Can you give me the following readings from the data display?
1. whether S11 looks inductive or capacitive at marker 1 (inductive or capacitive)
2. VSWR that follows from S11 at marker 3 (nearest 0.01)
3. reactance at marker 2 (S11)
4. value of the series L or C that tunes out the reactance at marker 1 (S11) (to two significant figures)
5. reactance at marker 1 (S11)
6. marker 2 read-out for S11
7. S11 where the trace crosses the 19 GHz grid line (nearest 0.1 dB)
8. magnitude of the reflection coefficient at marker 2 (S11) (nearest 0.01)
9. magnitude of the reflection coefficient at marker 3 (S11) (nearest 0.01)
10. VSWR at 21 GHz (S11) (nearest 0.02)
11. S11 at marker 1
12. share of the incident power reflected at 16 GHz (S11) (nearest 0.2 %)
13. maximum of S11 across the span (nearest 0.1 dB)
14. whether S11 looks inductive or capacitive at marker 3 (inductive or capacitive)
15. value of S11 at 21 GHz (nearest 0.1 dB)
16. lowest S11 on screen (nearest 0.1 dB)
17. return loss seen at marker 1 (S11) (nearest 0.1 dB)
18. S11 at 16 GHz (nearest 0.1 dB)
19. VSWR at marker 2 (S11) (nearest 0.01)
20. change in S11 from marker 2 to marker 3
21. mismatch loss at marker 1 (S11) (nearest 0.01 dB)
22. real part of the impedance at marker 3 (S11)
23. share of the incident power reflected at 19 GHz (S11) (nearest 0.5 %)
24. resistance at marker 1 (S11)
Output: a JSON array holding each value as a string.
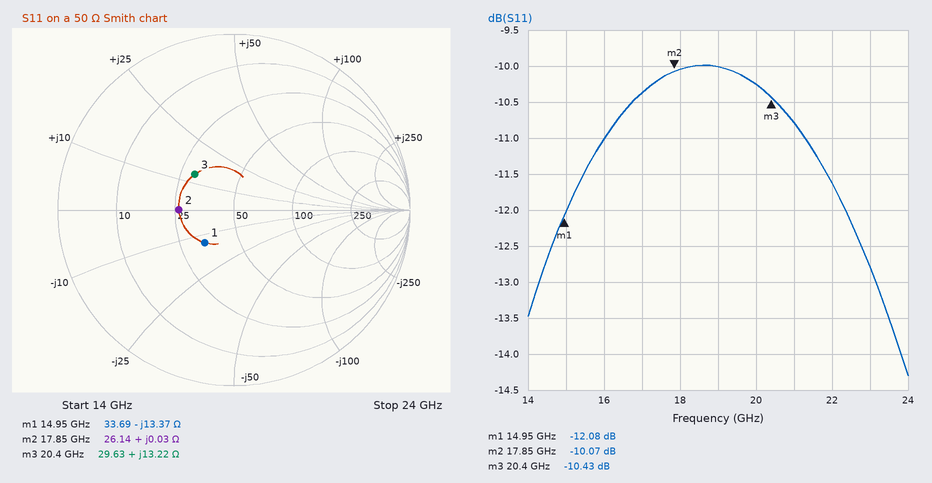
["capacitive", "1.86", "+0.03 Ω", "140 pH", "-13.37 Ω", "-10.07 dB", "-10.0 dB", "0.31", "0.30", "1.82", "-12.08 dB", "8.0 %", "-10.0 dB", "inductive", "-10.8 dB", "-14.3 dB", "12.1 dB", "-11.0 dB", "1.91", "-0.36 dB", "0.28 dB", "29.63 Ω", "10.0 %", "33.69 Ω"]
